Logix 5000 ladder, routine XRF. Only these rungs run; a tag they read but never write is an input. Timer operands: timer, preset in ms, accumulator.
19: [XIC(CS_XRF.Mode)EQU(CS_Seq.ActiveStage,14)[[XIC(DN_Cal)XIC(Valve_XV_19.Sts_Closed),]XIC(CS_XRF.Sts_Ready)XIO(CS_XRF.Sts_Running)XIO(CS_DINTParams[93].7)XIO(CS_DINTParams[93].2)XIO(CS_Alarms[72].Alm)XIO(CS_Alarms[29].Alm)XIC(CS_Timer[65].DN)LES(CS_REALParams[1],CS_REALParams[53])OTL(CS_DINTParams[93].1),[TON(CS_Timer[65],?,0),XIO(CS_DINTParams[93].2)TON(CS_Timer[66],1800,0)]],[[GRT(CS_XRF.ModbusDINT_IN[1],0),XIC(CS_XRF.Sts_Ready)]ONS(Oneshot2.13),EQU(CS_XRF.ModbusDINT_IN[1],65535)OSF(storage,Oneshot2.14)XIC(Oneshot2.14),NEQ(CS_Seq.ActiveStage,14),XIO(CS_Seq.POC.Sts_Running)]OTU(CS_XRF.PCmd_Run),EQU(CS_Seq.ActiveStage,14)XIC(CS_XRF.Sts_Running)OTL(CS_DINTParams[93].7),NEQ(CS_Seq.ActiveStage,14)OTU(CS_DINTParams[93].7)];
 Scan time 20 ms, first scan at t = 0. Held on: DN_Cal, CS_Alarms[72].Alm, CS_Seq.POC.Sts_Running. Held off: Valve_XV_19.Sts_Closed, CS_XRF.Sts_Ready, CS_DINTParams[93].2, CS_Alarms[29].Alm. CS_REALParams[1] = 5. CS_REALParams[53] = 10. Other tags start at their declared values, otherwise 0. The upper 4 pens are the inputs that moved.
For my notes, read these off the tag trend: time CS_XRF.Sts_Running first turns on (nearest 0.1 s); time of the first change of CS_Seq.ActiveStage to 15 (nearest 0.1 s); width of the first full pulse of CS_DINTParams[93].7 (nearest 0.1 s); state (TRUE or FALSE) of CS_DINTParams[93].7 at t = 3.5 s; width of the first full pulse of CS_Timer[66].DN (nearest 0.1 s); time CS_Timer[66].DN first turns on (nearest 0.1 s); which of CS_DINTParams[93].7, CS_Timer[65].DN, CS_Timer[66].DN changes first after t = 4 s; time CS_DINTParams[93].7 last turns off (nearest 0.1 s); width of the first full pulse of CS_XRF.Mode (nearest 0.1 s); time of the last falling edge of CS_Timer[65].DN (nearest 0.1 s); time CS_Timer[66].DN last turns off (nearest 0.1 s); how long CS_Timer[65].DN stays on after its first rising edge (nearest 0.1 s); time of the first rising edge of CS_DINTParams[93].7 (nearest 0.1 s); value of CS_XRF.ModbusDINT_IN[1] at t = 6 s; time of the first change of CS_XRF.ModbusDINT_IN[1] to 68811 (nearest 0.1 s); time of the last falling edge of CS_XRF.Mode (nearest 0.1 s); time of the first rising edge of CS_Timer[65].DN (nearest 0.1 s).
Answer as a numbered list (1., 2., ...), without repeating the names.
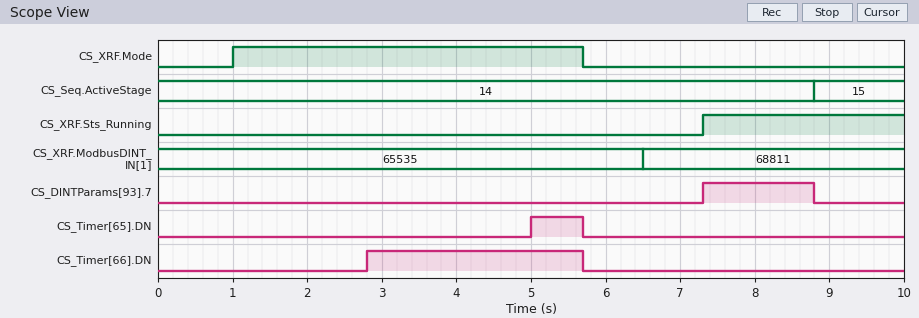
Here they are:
1. 7.3 s
2. 8.8 s
3. 1.5 s
4. FALSE
5. 2.9 s
6. 2.8 s
7. CS_Timer[65].DN
8. 8.8 s
9. 4.7 s
10. 5.7 s
11. 5.7 s
12. 0.7 s
13. 7.3 s
14. 65535
15. 6.5 s
16. 5.7 s
17. 5.0 s
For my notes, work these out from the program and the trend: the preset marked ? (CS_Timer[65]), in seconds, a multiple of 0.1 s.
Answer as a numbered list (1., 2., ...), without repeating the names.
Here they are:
1. 4.0 s
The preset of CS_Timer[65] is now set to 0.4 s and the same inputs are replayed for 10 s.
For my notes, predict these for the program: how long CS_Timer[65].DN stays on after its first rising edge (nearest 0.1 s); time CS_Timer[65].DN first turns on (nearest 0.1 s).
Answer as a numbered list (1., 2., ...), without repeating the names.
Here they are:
1. 4.3 s
2. 1.4 s
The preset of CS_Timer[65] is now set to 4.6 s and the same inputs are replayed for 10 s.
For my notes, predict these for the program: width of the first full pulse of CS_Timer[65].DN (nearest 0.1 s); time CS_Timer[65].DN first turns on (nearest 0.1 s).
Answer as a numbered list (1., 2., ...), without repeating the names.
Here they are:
1. 0.1 s
2. 5.6 s
